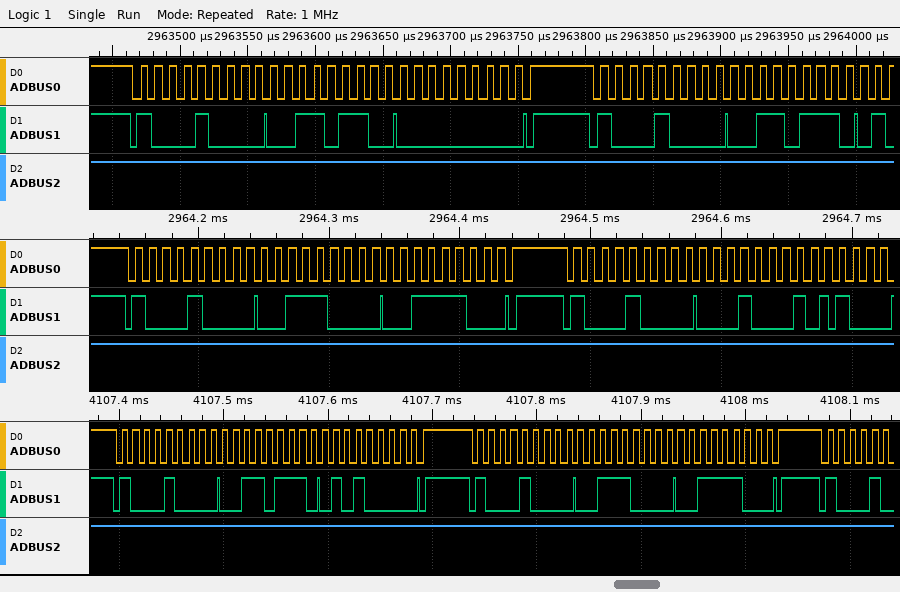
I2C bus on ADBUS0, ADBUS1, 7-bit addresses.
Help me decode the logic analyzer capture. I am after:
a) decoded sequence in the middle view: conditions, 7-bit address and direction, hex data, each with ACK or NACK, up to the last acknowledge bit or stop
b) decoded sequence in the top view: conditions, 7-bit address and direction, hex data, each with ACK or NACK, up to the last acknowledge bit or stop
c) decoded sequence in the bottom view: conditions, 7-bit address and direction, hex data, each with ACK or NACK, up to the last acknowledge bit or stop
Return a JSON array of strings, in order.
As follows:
["start, address 44 write ACK, 38 ACK, 3C ACK, stop, start, address 44 write ACK, 11 ACK", "start, address 44 write ACK, 36 ACK, 00 ACK, stop, start, address 44 write ACK, 37 ACK", "start, address 44 write ACK, 37 ACK, 50 ACK, stop, start, address 44 write ACK, 38 ACK, 3C ACK, stop"]
